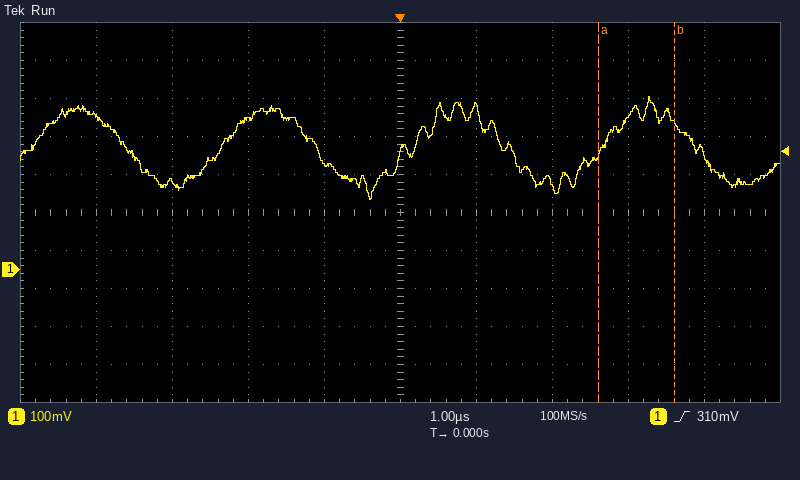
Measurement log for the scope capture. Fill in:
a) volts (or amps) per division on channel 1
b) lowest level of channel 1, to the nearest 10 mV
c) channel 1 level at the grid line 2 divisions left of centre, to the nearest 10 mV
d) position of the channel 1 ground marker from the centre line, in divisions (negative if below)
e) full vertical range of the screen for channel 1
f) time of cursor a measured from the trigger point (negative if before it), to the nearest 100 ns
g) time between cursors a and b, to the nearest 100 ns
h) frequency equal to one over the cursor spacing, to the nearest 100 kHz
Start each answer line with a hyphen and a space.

- 100 mV
- 180 mV
- 390 mV
- -1.5 div
- 1 V
- +2.6 µs
- 1.0 µs
- 1.0 MHz
